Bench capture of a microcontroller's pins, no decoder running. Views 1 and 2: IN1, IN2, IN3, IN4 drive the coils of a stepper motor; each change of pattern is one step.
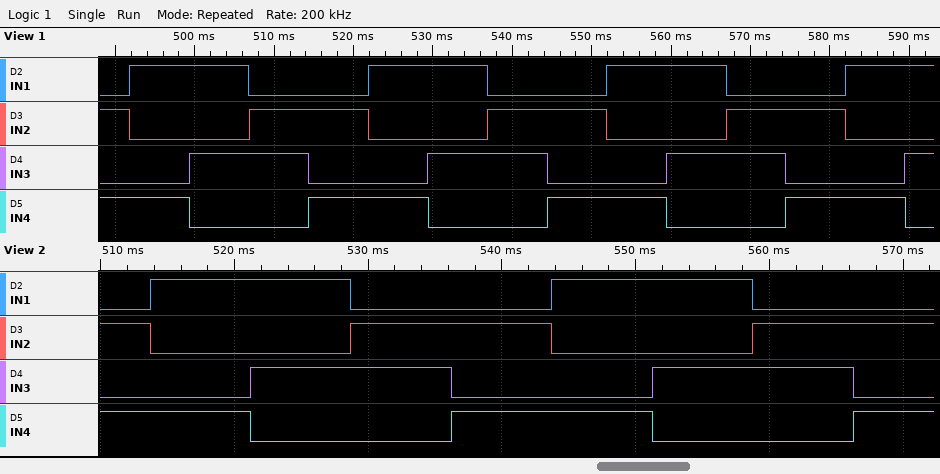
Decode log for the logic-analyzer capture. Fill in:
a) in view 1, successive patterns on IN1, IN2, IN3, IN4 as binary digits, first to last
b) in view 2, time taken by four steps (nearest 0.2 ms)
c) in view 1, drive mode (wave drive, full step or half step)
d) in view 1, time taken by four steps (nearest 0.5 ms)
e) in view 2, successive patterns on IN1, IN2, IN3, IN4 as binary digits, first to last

0101 1001 1010 0110 0101 1001 1010 0110 0101 1001 1010 0110 0101 1001 1010
30.0 ms
full step
30.0 ms
0101 1001 1010 0110 0101 1001 1010 0110 0101
